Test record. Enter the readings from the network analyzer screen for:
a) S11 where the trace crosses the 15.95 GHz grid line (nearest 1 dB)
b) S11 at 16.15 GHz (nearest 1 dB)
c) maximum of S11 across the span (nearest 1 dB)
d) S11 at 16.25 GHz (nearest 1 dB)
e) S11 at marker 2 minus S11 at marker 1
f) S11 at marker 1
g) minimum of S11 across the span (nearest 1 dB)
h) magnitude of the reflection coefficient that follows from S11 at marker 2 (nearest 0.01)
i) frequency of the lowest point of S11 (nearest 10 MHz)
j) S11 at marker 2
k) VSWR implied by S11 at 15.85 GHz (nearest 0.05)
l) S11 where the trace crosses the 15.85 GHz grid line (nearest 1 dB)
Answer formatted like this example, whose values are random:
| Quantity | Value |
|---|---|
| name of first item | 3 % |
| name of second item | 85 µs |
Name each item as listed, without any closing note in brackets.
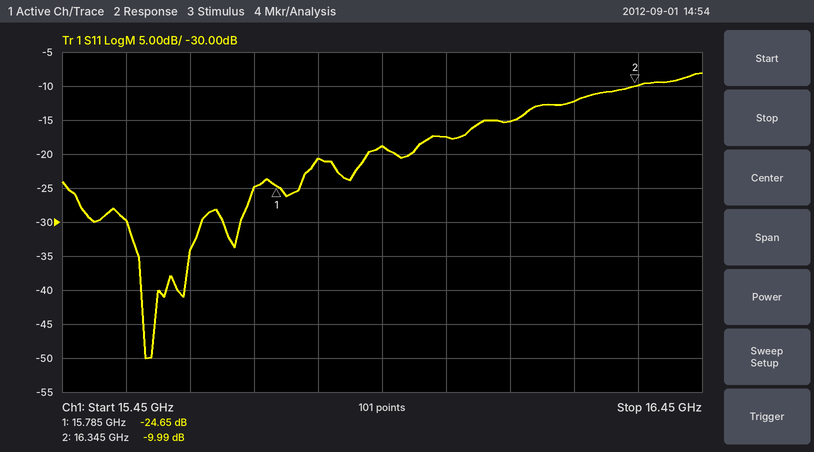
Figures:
| Quantity | Value |
|---|---|
| S11 where the trace crosses the 15.95 GHz grid line | -19 dB |
| S11 at 16.15 GHz | -15 dB |
| maximum of S11 across the span | -8 dB |
| S11 at 16.25 GHz | -12 dB |
| S11 at marker 2 minus S11 at marker 1 | 14.66 dB |
| S11 at marker 1 | -24.65 dB |
| minimum of S11 across the span | -50 dB |
| magnitude of the reflection coefficient that follows from S11 at marker 2 | 0.32 |
| frequency of the lowest point of S11 | 15.58 GHz |
| S11 at marker 2 | -9.99 dB |
| VSWR implied by S11 at 15.85 GHz | 1.20 |
| S11 where the trace crosses the 15.85 GHz grid line | -21 dB |
